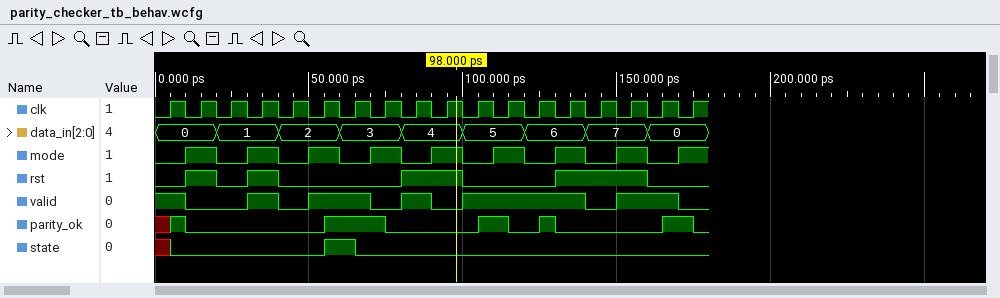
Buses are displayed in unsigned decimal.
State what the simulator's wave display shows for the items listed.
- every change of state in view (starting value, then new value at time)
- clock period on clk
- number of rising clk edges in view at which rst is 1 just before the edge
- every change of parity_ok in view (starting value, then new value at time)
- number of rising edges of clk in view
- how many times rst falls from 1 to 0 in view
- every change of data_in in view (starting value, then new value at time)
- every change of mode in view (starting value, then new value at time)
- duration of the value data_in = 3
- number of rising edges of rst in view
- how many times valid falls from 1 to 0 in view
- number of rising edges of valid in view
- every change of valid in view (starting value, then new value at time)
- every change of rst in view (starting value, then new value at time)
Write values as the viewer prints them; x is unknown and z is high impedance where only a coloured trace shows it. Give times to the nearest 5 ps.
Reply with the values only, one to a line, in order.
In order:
x, 0 at 5 ps, 1 at 55 ps, 0 at 65 ps
10 ps
7
x, 1 at 5 ps, 0 at 10 ps, 1 at 55 ps, 0 at 75 ps, 1 at 105 ps, 0 at 115 ps, 1 at 125 ps, 0 at 130 ps, 1 at 165 ps, 0 at 175 ps
18
4
0, 1 at 20 ps, 2 at 40 ps, 3 at 60 ps, 4 at 80 ps, 5 at 100 ps, 6 at 120 ps, 7 at 140 ps, 0 at 160 ps
0, 1 at 10 ps, 0 at 20 ps, 1 at 30 ps, 0 at 40 ps, 1 at 50 ps, 0 at 60 ps, 1 at 70 ps, 0 at 80 ps, 1 at 90 ps, 0 at 100 ps, 1 at 110 ps, 0 at 120 ps, 1 at 130 ps, 0 at 140 ps, 1 at 150 ps, 0 at 160 ps, 1 at 170 ps
20 ps
4
6
5
1, 0 at 10 ps, 1 at 30 ps, 0 at 40 ps, 1 at 50 ps, 0 at 70 ps, 1 at 80 ps, 0 at 90 ps, 1 at 100 ps, 0 at 140 ps, 1 at 150 ps, 0 at 170 ps
0, 1 at 10 ps, 0 at 20 ps, 1 at 30 ps, 0 at 40 ps, 1 at 80 ps, 0 at 100 ps, 1 at 130 ps, 0 at 160 ps
